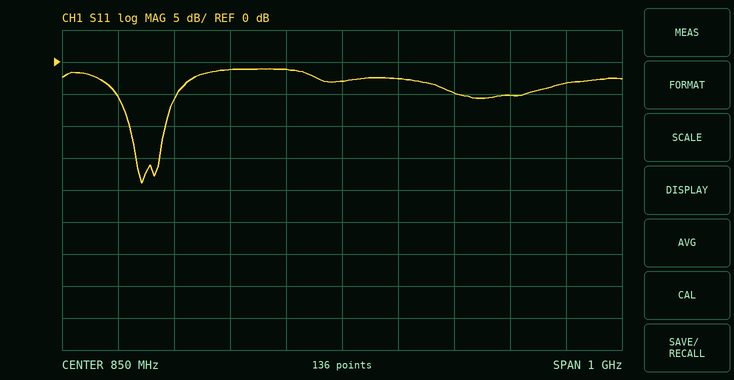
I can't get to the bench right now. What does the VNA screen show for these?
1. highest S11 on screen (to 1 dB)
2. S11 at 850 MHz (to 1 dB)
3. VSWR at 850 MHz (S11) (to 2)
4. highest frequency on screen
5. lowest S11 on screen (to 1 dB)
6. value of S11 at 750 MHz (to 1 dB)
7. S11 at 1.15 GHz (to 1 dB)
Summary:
-1 dB
-3 dB
6
1.35 GHz
-19 dB
-1 dB
-5 dB
